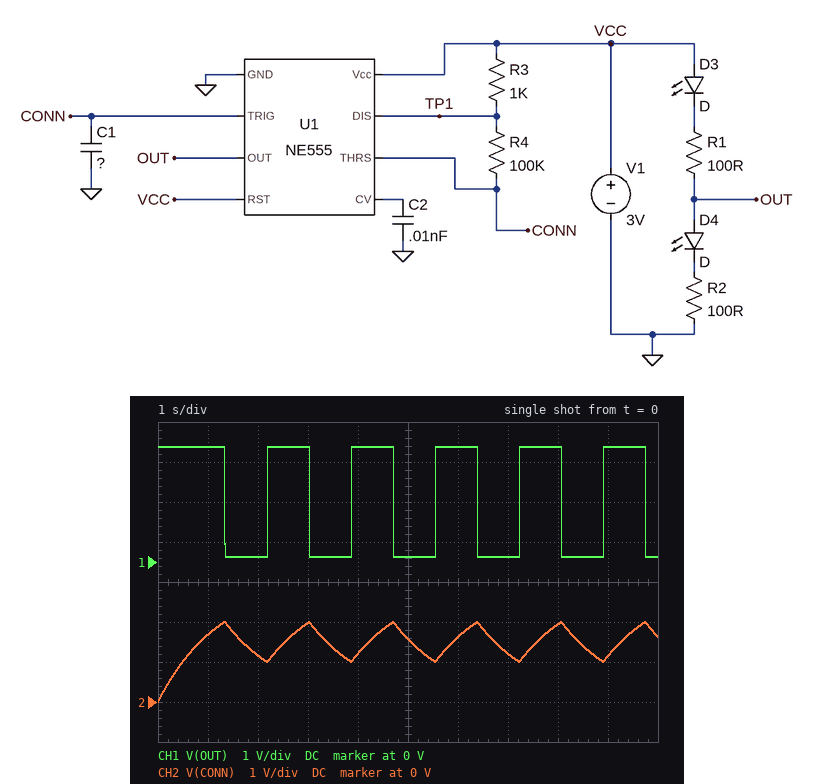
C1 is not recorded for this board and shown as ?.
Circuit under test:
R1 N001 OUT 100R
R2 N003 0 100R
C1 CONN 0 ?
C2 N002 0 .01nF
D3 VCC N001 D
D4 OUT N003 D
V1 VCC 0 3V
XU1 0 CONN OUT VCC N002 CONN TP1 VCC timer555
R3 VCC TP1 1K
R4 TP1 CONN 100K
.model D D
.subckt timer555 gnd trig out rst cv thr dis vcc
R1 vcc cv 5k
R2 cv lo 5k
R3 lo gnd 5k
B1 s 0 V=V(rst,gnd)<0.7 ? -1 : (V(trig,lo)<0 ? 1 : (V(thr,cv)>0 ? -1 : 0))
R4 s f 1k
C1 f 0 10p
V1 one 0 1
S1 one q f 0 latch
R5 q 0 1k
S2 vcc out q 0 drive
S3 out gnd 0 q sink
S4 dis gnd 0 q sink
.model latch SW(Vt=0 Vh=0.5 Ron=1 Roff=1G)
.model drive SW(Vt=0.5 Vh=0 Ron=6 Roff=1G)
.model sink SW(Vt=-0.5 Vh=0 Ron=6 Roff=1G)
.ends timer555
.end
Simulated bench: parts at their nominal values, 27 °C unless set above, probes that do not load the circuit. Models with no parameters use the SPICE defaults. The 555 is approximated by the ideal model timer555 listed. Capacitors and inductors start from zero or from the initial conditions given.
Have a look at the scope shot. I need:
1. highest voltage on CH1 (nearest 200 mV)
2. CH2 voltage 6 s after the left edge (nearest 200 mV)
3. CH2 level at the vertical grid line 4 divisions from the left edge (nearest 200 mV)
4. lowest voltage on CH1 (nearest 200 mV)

2.8 V
1.6 V
1.2 V
200 mV
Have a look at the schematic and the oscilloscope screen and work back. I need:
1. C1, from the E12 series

12 µF
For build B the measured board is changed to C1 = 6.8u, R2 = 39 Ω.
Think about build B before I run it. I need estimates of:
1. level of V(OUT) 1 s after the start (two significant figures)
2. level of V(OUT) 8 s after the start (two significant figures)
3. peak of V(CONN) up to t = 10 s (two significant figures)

130 mV
2.7 V
2.0 V
